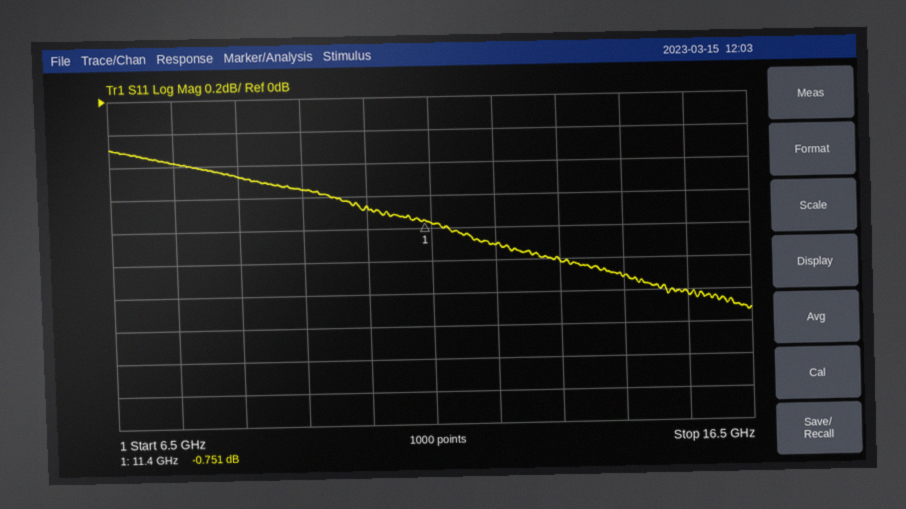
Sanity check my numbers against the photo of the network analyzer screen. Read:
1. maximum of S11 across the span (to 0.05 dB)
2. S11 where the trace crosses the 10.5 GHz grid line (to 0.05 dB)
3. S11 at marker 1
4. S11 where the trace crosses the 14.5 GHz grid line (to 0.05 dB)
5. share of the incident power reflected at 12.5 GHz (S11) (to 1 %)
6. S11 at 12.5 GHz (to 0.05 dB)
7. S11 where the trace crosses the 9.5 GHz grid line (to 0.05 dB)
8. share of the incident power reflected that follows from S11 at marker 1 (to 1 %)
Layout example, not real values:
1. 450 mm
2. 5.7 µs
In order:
1. -0.30 dB
2. -0.65 dB
3. -0.751 dB
4. -1.10 dB
5. 81 %
6. -0.90 dB
7. -0.55 dB
8. 84 %
